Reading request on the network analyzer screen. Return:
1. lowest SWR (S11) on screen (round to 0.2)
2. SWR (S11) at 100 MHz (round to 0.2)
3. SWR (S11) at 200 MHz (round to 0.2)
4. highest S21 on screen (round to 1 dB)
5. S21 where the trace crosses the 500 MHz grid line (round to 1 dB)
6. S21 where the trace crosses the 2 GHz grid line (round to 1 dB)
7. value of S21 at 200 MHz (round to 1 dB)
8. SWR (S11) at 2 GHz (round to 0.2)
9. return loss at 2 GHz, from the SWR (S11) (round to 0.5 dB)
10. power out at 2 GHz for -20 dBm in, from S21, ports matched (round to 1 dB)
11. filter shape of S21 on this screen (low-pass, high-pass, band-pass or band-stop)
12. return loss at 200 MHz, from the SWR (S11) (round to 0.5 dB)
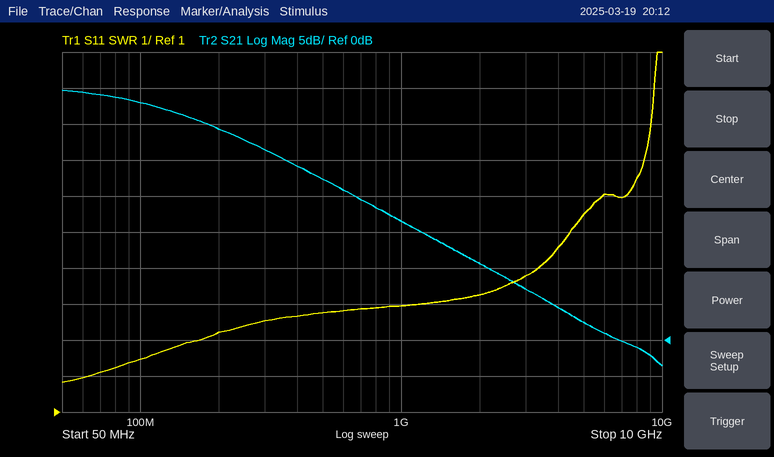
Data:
1.8
2.4
3.2
35 dB
22 dB
11 dB
29 dB
4.2
4.0 dB
-9 dBm
low-pass
5.5 dB
